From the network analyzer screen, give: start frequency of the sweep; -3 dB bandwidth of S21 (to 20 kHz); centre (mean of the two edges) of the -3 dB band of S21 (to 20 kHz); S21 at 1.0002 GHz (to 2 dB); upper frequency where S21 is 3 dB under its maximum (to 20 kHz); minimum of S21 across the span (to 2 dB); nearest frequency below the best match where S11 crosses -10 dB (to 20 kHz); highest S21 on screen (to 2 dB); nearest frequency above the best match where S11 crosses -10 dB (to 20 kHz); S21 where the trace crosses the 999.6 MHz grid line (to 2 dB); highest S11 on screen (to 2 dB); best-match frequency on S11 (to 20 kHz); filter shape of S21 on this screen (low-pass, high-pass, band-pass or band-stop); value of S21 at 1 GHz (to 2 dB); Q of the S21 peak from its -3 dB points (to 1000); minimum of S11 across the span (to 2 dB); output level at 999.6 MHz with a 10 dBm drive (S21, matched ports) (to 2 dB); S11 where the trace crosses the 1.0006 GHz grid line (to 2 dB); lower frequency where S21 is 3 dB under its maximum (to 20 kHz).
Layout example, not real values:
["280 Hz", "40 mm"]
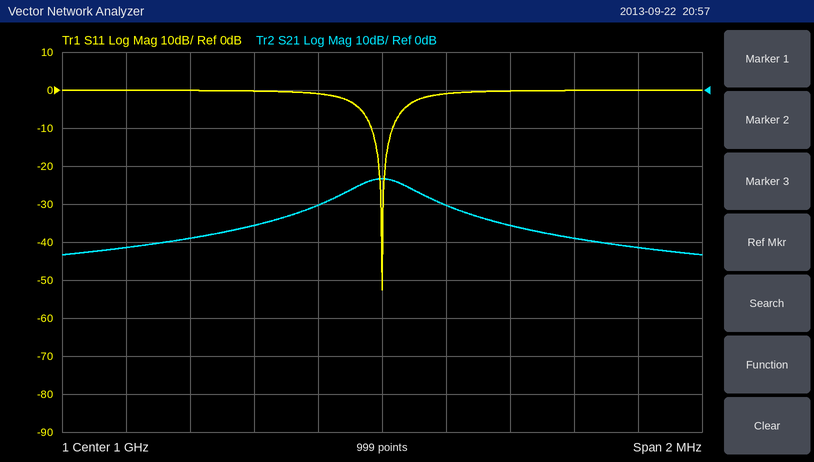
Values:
["999 MHz", "200 kHz", "1.00000 GHz", "-30 dB", "1.00010 GHz", "-44 dB", "999.96 MHz", "-24 dB", "1.00004 GHz", "-36 dB", "0 dB", "1.00000 GHz", "band-pass", "-24 dB", "5000", "-52 dB", "-26 dBm", "0 dB", "999.90 MHz"]
